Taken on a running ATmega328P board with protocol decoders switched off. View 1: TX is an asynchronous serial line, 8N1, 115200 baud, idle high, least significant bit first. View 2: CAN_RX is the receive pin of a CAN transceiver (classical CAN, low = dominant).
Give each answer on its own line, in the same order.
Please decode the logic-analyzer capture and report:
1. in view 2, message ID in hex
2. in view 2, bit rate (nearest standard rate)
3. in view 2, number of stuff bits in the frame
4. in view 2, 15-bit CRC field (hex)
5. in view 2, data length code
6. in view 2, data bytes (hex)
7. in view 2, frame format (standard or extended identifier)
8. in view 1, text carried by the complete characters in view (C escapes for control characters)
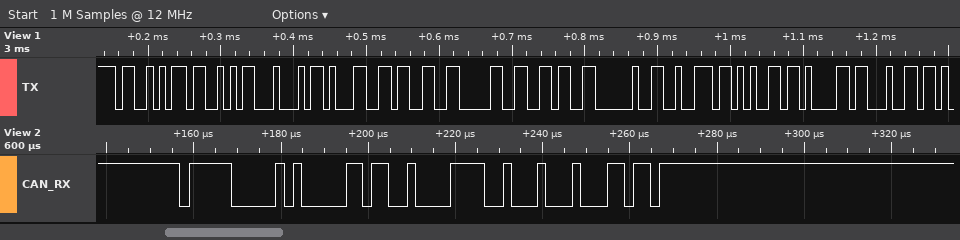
0x7C1
500 kbit/s
3
0x088D
2
C8 79
standard
"SSD1306 read"
